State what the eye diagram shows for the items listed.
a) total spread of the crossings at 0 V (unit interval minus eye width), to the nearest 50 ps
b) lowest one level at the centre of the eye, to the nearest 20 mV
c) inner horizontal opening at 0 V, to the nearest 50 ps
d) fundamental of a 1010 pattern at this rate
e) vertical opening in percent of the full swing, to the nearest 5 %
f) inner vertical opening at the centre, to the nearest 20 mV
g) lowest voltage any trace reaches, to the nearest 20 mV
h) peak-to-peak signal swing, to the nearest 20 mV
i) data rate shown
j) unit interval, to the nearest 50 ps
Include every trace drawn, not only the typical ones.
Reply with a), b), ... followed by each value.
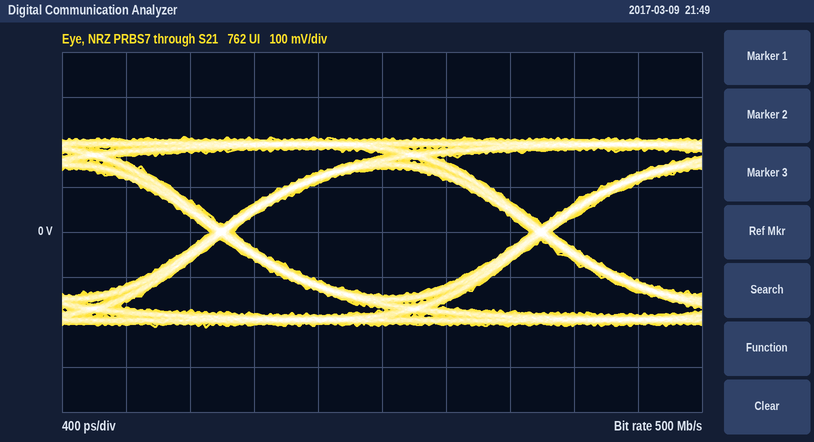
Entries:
a) 150 ps
b) 140 mV
c) 1.85 ns
d) 250 MHz
e) 65 %
f) 280 mV
g) -220 mV
h) 420 mV
i) 500 Mb/s
j) 2.00 ns
